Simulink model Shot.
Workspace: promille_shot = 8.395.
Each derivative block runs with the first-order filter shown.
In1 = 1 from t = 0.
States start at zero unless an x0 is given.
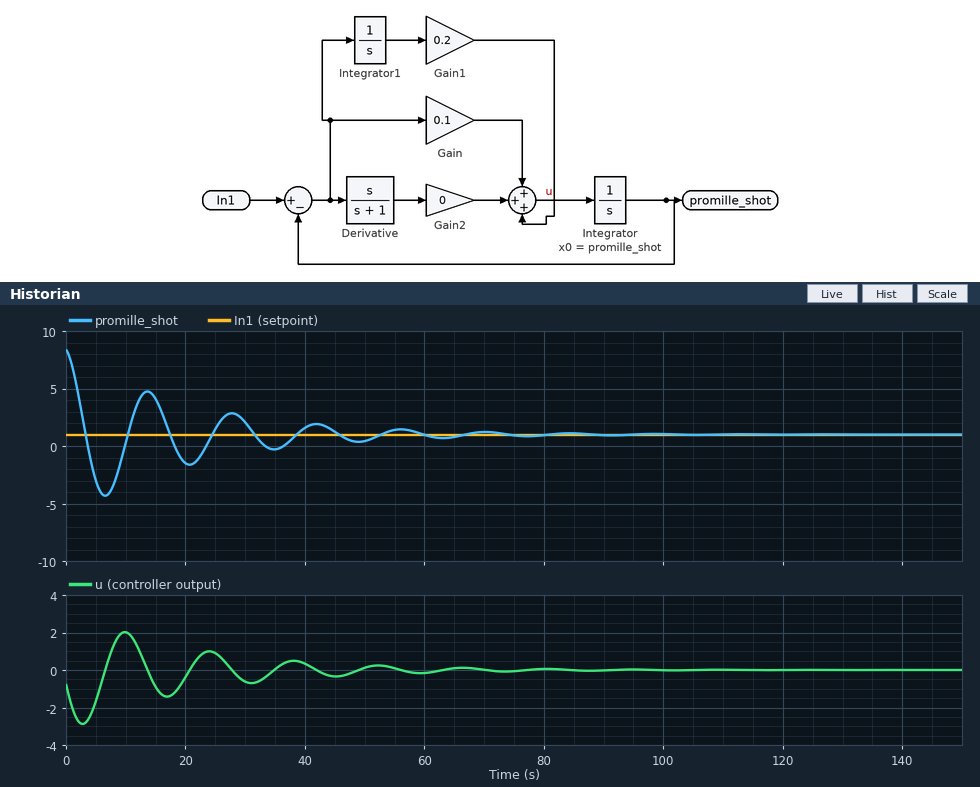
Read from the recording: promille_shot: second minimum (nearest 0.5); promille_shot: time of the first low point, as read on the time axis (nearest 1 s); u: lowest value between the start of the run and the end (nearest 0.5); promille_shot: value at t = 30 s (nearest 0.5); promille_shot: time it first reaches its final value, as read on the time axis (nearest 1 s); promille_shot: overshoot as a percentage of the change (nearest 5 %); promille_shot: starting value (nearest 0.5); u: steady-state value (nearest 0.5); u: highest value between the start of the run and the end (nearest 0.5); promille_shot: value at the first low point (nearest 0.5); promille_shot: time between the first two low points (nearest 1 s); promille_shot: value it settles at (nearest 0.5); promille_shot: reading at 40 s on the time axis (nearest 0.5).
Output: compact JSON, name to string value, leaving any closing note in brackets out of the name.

{"promille_shot: second minimum": "-1.5", "promille_shot: time of the first low point, as read on the time axis": "7 s", "u: lowest value between the start of the run and the end": "-3.0", "promille_shot: value at t = 30 s": "2.0", "promille_shot: time it first reaches its final value, as read on the time axis": "3 s", "promille_shot: overshoot as a percentage of the change": "70 %", "promille_shot: starting value": "8.5", "u: steady-state value": "0.0", "u: highest value between the start of the run and the end": "2.0", "promille_shot: value at the first low point": "-4.5", "promille_shot: time between the first two low points": "14 s", "promille_shot: value it settles at": "1.0", "promille_shot: reading at 40 s on the time axis": "1.5"}
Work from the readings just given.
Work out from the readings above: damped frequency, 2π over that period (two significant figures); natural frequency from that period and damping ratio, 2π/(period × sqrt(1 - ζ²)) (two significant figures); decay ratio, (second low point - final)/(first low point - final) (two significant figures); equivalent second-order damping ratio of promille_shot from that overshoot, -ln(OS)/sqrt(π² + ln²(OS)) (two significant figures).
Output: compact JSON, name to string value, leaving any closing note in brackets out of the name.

{"damped frequency, 2π over that period": "0.45 rad/s", "natural frequency from that period and damping ratio, 2π/(period × sqrt(1 - ζ²))": "0.45 rad/s", "decay ratio, (second low point - final)/(first low point - final)": "0.45", "equivalent second-order damping ratio of promille_shot from that overshoot, -ln(OS)/sqrt(π² + ln²(OS))": "0.11"}
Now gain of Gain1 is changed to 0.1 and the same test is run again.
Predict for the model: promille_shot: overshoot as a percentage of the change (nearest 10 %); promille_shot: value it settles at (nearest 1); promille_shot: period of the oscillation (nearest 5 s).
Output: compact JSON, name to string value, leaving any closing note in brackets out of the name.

{"promille_shot: overshoot as a percentage of the change": "60 %", "promille_shot: value it settles at": "1", "promille_shot: period of the oscillation": "20 s"}
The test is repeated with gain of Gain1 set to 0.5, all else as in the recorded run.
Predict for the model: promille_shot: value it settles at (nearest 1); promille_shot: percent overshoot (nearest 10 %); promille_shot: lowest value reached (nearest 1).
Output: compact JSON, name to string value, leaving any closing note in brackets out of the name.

{"promille_shot: value it settles at": "1", "promille_shot: percent overshoot": "80 %", "promille_shot: lowest value reached": "-5"}
